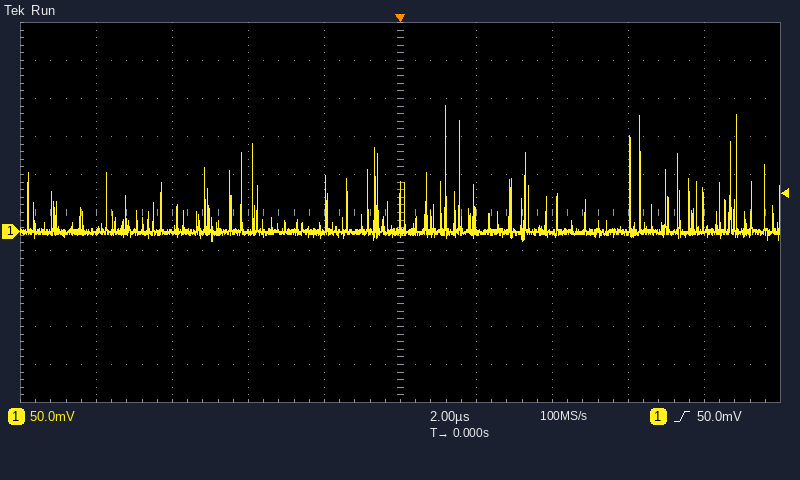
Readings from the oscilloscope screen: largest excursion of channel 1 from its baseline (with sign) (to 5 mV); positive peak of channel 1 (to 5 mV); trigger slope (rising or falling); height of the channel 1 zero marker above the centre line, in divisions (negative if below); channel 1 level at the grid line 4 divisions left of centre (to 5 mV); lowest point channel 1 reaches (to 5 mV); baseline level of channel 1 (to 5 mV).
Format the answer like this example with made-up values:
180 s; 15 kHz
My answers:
+165 mV; 165 mV; rising; -0.5 div; 0 mV; -10 mV; 0 mV
